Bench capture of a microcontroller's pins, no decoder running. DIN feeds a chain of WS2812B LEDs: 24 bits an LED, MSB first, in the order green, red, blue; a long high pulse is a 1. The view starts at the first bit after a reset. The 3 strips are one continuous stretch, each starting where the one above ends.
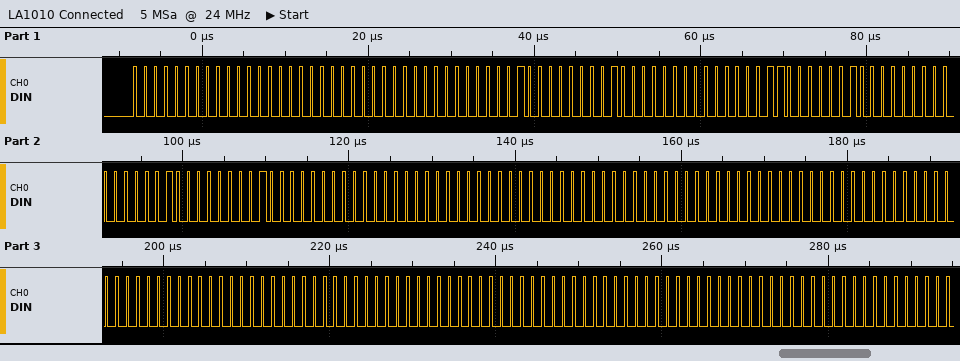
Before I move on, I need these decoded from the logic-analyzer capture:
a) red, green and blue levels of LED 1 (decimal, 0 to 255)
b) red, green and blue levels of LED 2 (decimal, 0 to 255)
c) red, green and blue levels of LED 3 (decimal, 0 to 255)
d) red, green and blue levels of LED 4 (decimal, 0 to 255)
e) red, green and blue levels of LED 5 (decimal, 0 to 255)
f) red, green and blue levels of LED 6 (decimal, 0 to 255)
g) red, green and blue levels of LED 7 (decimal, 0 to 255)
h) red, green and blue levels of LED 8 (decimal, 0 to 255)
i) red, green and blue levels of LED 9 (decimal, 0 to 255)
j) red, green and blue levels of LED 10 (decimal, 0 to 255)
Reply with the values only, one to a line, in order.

0, 0, 0
4, 0, 2
6, 0, 4
4, 0, 2
0, 0, 0
0, 0, 0
0, 0, 0
0, 0, 0
0, 0, 0
0, 0, 0
